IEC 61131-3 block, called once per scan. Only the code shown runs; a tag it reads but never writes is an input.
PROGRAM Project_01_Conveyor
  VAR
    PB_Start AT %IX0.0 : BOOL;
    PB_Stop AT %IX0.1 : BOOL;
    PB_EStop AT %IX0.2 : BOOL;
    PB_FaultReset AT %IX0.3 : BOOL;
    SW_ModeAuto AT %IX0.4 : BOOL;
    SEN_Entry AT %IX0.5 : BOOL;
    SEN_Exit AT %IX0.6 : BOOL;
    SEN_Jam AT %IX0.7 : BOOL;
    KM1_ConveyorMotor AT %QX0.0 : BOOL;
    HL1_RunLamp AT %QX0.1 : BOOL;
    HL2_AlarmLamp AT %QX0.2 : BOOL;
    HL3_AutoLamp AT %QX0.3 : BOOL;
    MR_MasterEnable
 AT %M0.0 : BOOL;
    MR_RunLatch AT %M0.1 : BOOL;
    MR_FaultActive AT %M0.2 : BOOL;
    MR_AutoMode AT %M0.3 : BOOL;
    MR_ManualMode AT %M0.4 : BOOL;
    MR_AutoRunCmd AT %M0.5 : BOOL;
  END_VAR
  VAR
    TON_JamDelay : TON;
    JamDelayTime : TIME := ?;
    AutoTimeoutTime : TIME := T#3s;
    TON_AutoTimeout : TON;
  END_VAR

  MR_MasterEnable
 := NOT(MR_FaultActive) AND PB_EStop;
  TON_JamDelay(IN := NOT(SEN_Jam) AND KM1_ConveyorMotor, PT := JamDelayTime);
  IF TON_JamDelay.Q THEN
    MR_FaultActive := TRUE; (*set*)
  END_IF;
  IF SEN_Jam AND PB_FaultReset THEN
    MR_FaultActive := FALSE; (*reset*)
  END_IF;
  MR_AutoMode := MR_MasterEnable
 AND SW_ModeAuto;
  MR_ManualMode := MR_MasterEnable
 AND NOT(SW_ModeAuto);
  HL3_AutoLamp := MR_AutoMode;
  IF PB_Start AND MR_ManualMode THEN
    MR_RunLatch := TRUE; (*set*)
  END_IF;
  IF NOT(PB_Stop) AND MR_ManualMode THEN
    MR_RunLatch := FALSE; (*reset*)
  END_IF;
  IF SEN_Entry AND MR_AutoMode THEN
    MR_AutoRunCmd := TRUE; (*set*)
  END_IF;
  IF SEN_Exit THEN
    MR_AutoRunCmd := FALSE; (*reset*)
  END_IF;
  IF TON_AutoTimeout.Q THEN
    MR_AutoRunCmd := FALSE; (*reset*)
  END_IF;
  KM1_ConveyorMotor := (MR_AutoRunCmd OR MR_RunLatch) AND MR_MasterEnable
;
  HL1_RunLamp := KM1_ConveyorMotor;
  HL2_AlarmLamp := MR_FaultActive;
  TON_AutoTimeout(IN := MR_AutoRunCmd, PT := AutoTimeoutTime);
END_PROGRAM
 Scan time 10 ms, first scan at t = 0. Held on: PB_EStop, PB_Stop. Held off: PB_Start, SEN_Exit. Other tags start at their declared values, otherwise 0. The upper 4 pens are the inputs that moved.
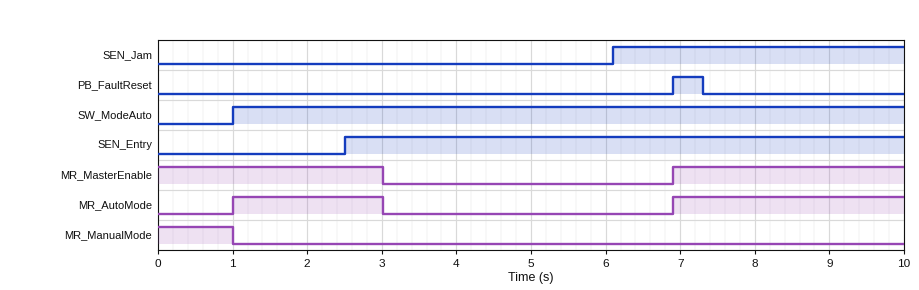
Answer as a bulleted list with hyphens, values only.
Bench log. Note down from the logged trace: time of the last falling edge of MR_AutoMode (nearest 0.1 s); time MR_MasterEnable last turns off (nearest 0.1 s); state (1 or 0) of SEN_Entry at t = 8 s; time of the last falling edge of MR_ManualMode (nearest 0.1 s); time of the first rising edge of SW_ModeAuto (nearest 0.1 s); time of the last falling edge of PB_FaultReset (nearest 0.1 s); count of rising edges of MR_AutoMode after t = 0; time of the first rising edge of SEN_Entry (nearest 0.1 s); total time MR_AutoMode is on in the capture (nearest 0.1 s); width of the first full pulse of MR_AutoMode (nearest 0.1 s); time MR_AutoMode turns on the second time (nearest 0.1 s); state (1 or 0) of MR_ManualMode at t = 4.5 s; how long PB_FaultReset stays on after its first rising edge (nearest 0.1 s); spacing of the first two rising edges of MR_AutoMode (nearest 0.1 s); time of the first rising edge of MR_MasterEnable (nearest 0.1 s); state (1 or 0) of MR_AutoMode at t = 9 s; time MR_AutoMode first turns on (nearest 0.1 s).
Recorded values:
- 3.0 s
- 3.0 s
- 1
- 1.0 s
- 1.0 s
- 7.3 s
- 2
- 2.5 s
- 5.1 s
- 2.0 s
- 6.9 s
- 0
- 0.4 s
- 5.9 s
- 6.9 s
- 1
- 1.0 s
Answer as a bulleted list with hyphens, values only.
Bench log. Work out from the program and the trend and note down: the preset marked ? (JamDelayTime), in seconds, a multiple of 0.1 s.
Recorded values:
- 0.5 s
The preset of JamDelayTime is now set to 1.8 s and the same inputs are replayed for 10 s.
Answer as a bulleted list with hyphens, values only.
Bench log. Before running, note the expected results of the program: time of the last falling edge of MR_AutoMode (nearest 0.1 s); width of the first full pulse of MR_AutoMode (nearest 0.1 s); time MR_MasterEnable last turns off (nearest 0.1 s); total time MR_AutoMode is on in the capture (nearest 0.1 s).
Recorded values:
- 4.3 s
- 3.3 s
- 4.3 s
- 6.4 s
